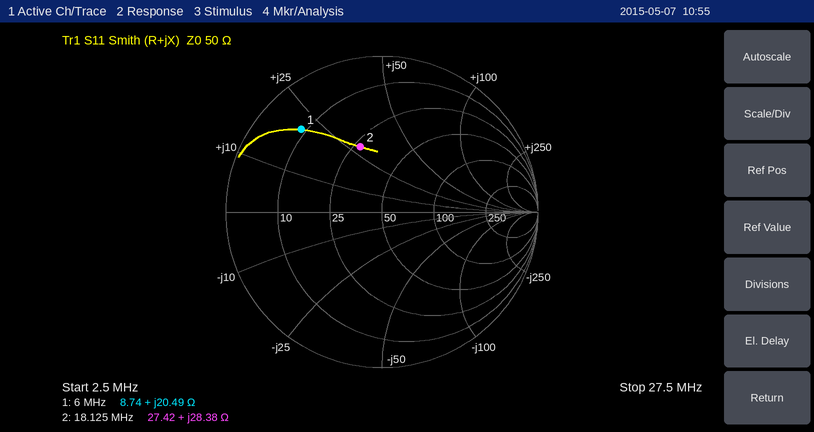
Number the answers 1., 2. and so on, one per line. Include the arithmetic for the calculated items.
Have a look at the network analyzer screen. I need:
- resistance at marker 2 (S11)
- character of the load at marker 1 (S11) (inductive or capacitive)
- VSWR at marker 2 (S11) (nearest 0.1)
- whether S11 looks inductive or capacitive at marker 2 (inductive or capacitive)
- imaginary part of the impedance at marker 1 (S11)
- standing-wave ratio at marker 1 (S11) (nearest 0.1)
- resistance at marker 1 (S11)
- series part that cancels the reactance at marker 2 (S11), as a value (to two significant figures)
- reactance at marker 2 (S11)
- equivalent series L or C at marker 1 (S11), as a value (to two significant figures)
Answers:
1. 27.42 Ω
2. inductive
3. 2.6
4. inductive
5. +20.49 Ω
6. 6.7
7. 8.74 Ω
8. C = 1/(2π × 18.125 MHz × 28.38 Ω) ≈ 309 pF, so 310 pF to two significant figures
9. +28.38 Ω
10. L = 20.49 Ω/(2π × 6 MHz) ≈ 544 nH, so 540 nH to two significant figures
